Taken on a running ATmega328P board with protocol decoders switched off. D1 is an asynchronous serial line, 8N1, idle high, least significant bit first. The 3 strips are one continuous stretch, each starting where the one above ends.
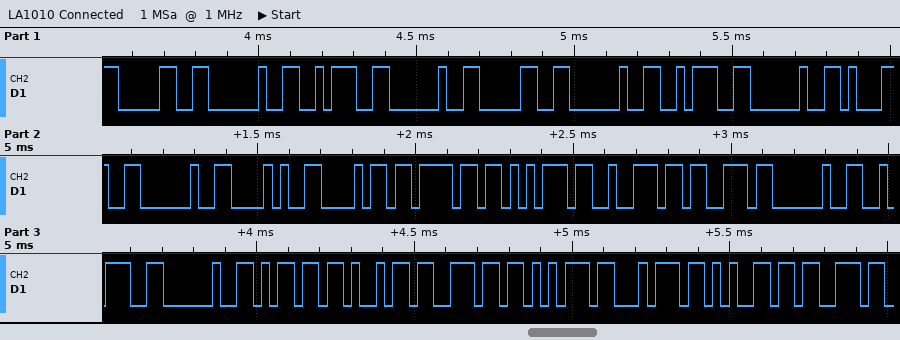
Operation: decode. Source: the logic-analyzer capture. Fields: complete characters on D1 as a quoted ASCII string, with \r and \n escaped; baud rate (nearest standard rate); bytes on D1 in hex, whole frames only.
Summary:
"0 : 0 : 1 (hours : minutes"
38400 baud
30 20 3A 20 30 20 3A 20 31 20 28 68 6F 75 72 73 20 3A 20 6D 69 6E 75 74 65 73
